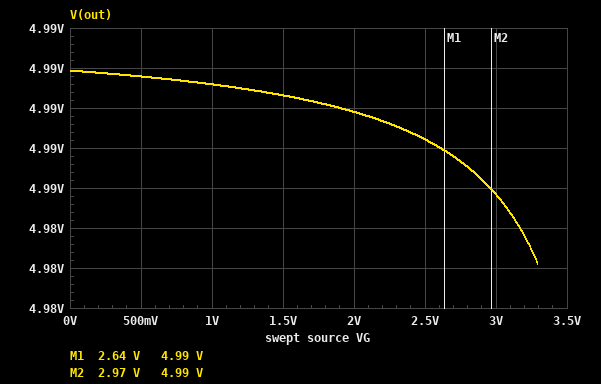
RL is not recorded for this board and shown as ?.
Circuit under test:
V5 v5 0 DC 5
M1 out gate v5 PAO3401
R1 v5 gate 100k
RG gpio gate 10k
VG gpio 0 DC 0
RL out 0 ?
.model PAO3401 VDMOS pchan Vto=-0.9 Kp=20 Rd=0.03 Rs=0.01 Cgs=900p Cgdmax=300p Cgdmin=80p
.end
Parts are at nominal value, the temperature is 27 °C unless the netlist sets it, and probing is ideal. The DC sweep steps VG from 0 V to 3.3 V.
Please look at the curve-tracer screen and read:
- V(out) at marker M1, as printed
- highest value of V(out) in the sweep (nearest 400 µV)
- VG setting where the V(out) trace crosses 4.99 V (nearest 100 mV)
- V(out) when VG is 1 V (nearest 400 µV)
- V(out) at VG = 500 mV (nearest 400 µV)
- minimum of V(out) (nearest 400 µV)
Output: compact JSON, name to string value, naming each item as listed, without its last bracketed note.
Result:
{"V(out) at marker M1, as printed": "4.99 V", "highest value of V(out) in the sweep": "4.9920 V", "VG setting where the V(out) trace crosses 4.99 V": "2.6 V", "V(out) when VG is 1 V": "4.9912 V", "V(out) at VG = 500 mV": "4.9916 V", "minimum of V(out)": "4.9820 V"}
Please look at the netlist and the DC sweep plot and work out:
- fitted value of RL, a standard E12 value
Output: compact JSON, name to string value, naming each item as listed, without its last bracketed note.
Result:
{"fitted value of RL, a standard E12 value": "33 Ω"}
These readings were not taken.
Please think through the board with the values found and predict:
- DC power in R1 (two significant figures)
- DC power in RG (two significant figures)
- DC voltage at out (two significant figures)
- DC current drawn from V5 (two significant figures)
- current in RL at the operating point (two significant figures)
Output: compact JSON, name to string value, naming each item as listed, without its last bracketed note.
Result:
{"DC power in R1": "210 µW", "DC power in RG": "21 µW", "DC voltage at out": "5.0 V", "DC current drawn from V5": "150 mA", "current in RL at the operating point": "150 mA"}
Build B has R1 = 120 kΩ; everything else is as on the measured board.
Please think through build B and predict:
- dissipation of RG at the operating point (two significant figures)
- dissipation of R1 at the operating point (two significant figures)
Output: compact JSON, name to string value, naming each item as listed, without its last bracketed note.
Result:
{"dissipation of RG at the operating point": "15 µW", "dissipation of R1 at the operating point": "180 µW"}
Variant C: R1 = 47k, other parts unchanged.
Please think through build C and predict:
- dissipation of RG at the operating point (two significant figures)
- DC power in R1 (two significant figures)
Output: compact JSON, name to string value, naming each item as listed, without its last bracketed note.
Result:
{"dissipation of RG at the operating point": "77 µW", "DC power in R1": "360 µW"}
